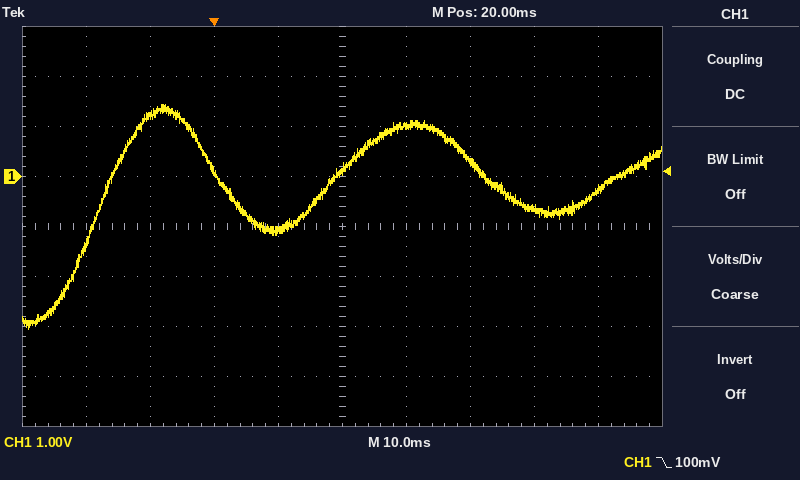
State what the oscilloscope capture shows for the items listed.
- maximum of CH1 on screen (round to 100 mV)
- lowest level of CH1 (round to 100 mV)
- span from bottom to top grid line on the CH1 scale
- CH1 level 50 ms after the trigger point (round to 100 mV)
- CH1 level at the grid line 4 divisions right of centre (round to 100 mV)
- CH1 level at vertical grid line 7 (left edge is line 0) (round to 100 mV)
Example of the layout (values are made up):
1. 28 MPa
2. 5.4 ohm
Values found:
1. 1.4 V
2. -3.0 V
3. 8 V
4. -600 mV
5. -300 mV
6. 300 mV
